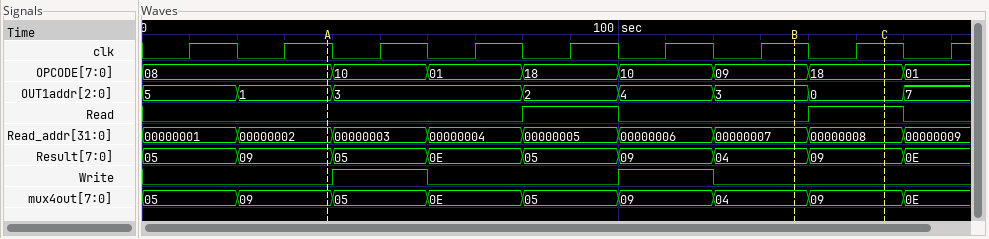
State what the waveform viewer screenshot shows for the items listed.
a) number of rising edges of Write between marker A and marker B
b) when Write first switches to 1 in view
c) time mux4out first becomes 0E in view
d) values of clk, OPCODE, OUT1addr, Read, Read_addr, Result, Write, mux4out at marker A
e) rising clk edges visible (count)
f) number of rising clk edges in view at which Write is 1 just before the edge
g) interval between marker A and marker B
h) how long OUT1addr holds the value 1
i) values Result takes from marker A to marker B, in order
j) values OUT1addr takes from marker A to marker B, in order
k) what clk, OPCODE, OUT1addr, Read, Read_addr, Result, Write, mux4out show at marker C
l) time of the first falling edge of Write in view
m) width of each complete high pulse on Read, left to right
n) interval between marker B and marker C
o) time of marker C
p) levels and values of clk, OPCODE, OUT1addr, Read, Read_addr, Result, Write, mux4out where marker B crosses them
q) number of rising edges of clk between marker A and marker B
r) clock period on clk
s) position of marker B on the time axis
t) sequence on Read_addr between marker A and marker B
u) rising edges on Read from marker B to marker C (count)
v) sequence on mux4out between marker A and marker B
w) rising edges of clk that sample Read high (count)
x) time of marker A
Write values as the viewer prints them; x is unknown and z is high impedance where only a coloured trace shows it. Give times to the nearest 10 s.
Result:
2
40 s
60 s
clk=1, OPCODE=08, OUT1addr=1, Read=0, Read_addr=00000002, Result=09, Write=0, mux4out=09
9
2
100 s
20 s
09, 05, 0E, 05, 09, 04
1, 3, 2, 4, 3
clk=1, OPCODE=18, OUT1addr=0, Read=1, Read_addr=00000008, Result=09, Write=0, mux4out=09
60 s
20 s, 20 s
20 s
160 s
clk=1, OPCODE=09, OUT1addr=3, Read=0, Read_addr=00000007, Result=04, Write=0, mux4out=04
5
20 s
140 s
00000002, 00000003, 00000004, 00000005, 00000006, 00000007
1
09, 05, 0E, 05, 09, 04
2
40 s
